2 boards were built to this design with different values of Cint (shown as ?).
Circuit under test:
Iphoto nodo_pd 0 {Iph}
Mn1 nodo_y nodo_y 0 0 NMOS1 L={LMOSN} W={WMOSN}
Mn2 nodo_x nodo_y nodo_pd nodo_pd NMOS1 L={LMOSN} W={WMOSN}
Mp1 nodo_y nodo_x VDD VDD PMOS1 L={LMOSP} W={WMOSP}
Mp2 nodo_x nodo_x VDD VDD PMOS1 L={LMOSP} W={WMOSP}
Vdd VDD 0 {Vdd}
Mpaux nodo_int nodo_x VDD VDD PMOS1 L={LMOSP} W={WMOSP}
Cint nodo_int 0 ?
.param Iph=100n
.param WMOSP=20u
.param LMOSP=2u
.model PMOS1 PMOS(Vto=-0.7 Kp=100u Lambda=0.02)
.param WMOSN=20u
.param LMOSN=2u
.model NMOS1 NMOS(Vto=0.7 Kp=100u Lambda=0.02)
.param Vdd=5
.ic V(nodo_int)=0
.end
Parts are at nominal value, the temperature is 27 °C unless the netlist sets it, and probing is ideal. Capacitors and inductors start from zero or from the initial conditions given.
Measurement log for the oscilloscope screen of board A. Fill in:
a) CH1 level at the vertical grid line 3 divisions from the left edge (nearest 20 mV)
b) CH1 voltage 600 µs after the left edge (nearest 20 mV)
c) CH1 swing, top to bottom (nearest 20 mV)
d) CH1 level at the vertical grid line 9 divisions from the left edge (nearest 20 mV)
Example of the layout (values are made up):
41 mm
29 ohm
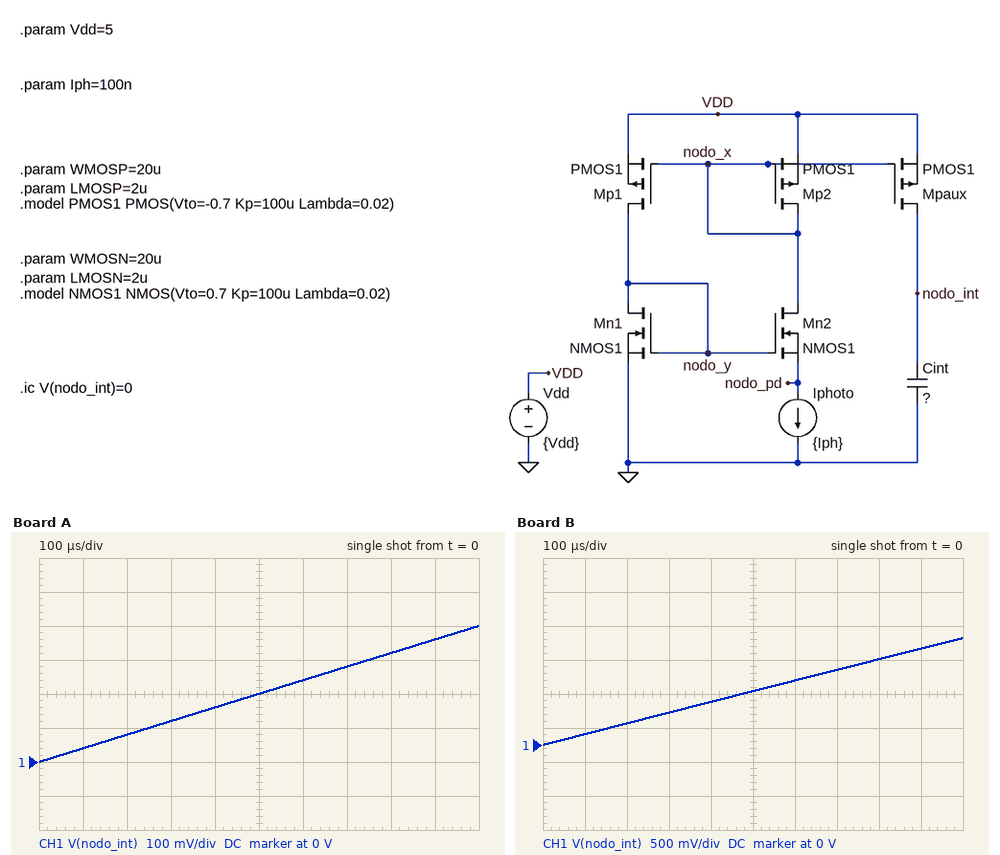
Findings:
120 mV
240 mV
400 mV
360 mV
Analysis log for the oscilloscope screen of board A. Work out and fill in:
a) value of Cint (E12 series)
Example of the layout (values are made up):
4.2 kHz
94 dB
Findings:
270 pF
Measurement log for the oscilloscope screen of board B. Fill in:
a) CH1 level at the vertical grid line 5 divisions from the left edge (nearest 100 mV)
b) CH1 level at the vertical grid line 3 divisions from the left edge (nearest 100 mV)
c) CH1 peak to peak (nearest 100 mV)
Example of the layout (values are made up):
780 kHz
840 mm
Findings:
800 mV
500 mV
1.6 V
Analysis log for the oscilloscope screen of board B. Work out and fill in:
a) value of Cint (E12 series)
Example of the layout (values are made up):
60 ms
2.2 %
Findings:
68 pF
